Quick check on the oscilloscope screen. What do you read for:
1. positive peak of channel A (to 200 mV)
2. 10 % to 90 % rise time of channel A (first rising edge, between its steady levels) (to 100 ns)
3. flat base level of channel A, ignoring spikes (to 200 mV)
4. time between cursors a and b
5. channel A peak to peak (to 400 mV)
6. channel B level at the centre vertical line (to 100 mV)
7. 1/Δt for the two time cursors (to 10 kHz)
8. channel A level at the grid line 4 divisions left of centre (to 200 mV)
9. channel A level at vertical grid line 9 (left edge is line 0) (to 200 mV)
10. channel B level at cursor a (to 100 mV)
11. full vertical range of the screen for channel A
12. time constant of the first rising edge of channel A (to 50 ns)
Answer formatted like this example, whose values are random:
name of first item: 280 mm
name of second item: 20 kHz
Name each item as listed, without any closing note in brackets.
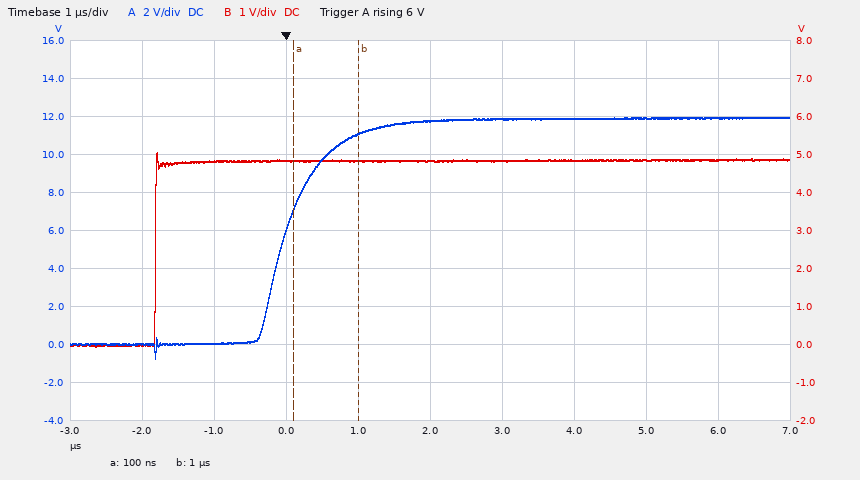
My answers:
positive peak of channel A: 12.0 V
10 % to 90 % rise time of channel A (first rising edge, between its steady levels): 1.1 µs
flat base level of channel A, ignoring spikes: 0.0 V
time between cursors a and b: 900 ns
channel A peak to peak: 12.8 V
channel B level at the centre vertical line: 4.8 V
1/Δt for the two time cursors: 1.11 MHz
channel A level at the grid line 4 divisions left of centre: 0.0 V
channel A level at vertical grid line 9 (left edge is line 0): 12.0 V
channel B level at cursor a: 4.8 V
full vertical range of the screen for channel A: 20 V
time constant of the first rising edge of channel A: 500 ns
